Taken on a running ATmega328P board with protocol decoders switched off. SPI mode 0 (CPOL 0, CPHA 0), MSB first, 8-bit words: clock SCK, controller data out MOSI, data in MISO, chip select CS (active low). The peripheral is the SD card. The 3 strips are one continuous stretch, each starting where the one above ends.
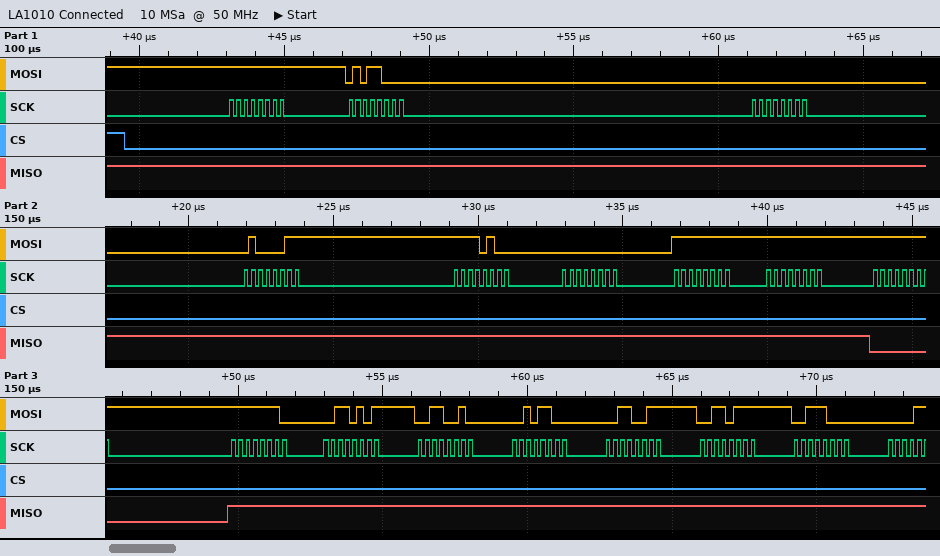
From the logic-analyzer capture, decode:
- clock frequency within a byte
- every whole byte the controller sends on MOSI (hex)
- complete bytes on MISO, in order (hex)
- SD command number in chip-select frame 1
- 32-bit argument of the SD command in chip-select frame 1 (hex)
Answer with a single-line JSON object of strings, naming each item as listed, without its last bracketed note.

{"clock frequency within a byte": "4 MHz", "every whole byte the controller sends on MOSI": "FF 58 00 43 F4 00 FF FF FF FE 35 32 2C 33 37 38", "complete bytes on MISO, in order": "FF FF FF FF FF FF FF FF 00 FF FF FF FF FF FF FF", "SD command number in chip-select frame 1": "CMD24", "32-bit argument of the SD command in chip-select frame 1": "0x0043F400"}
